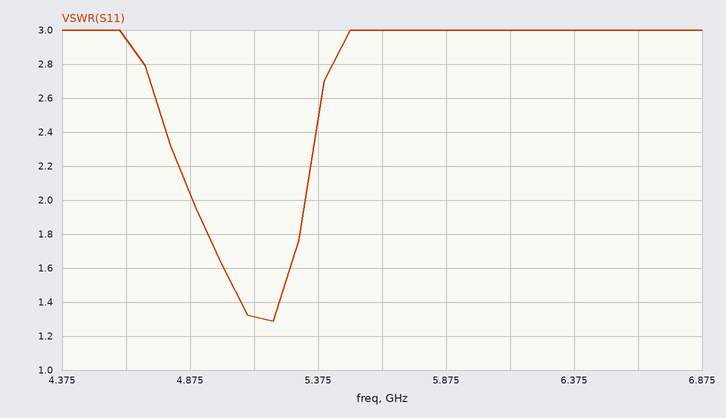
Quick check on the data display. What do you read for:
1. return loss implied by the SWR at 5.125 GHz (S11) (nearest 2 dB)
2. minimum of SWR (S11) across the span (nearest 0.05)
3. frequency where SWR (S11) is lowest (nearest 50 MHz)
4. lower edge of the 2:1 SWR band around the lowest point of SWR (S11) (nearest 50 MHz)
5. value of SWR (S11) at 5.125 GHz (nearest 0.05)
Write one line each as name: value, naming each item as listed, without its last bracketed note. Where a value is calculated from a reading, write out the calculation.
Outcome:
return loss implied by the SWR at 5.125 GHz (S11): −20 log10((1.3 − 1)/(1.3 + 1)) ≈ 18 dB
minimum of SWR (S11) across the span: 1.30
frequency where SWR (S11) is lowest: 5.20 GHz
lower edge of the 2:1 SWR band around the lowest point of SWR (S11): 4.90 GHz
value of SWR (S11) at 5.125 GHz: 1.30
